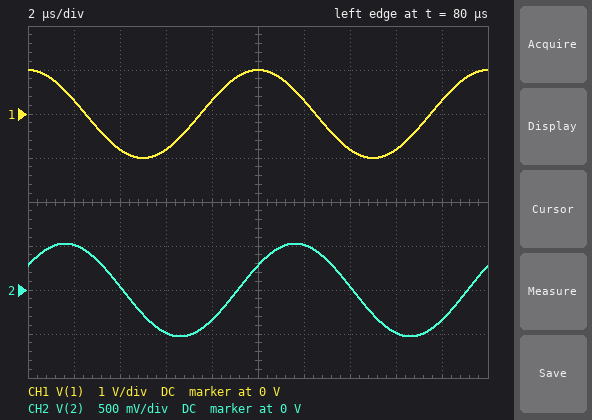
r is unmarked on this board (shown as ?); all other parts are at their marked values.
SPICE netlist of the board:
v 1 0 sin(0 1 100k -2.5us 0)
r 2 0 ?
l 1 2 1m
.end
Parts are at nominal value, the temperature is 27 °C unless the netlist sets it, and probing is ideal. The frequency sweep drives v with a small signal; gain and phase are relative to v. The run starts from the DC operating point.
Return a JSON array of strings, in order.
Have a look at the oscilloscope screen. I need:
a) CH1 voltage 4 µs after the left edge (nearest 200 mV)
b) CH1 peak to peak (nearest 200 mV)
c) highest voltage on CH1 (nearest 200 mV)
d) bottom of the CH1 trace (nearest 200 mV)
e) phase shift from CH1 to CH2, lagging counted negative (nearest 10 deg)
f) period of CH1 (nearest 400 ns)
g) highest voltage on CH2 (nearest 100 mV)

["-800 mV", "2.0 V", "1.0 V", "-1.0 V", "-60 deg", "10.0 µs", "500 mV"]
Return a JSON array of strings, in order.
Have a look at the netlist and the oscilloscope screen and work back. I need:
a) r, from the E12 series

["390 Ω"]
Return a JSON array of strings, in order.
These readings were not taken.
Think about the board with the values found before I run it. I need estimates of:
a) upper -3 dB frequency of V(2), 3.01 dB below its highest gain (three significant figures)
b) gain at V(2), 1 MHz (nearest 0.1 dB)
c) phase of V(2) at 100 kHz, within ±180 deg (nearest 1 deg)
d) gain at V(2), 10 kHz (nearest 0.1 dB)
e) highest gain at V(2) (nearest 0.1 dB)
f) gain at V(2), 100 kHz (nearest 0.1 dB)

["62.1 kHz", "-24.2 dB", "-58 deg", "-0.1 dB", "0 dB", "-5.6 dB"]
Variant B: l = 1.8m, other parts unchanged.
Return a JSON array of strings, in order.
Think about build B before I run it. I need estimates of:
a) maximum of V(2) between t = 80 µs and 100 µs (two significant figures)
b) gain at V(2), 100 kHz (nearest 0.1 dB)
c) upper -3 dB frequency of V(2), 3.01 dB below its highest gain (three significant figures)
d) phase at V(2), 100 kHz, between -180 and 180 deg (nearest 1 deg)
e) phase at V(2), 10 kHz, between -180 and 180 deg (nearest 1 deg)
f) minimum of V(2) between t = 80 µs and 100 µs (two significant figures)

["330 mV", "-9.7 dB", "34.5 kHz", "-71 deg", "-16 deg", "-330 mV"]
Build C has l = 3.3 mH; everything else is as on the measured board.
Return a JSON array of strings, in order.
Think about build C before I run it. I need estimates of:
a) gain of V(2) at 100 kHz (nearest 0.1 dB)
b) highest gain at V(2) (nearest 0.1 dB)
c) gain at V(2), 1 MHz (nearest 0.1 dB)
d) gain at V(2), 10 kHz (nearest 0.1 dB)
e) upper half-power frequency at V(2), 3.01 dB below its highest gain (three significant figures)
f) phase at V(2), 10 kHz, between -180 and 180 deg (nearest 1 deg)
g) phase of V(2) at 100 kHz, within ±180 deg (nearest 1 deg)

["-14.7 dB", "0 dB", "-34.5 dB", "-1.1 dB", "18.8 kHz", "-28 deg", "-79 deg"]
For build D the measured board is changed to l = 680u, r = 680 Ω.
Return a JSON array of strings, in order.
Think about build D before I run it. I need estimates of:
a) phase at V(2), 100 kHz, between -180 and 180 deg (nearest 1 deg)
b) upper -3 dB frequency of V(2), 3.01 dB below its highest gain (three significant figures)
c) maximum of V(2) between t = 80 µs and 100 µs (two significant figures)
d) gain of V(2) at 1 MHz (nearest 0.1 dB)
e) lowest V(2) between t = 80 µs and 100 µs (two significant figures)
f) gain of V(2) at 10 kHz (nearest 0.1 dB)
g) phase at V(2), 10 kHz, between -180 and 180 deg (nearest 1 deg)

["-32 deg", "159 kHz", "850 mV", "-16.1 dB", "-850 mV", "0 dB", "-4 deg"]
